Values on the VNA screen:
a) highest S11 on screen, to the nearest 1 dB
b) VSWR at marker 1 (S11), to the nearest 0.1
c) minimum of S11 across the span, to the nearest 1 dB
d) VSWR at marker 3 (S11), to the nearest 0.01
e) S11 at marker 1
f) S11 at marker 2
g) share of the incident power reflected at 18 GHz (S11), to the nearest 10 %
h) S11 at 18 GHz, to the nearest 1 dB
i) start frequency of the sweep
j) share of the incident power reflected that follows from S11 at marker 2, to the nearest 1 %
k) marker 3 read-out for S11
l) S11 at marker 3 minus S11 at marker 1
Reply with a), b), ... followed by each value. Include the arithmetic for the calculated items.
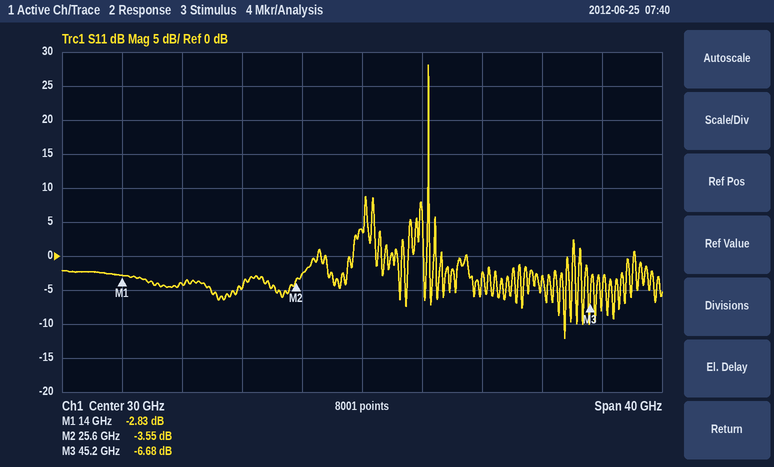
a) 28 dB
b) (1 + 0.7219)/(1 − 0.7219) ≈ 6.2
c) -12 dB
d) (1 + 0.4634)/(1 − 0.4634) ≈ 2.73
e) -2.83 dB
f) -3.55 dB
g) 10^(-4/10) ≈ 40 %
h) -4 dB
i) 10 GHz
j) 10^(-3.55/10) ≈ 44 %
k) -6.68 dB
l) -6.68 − (-2.83) = -3.85 dB
